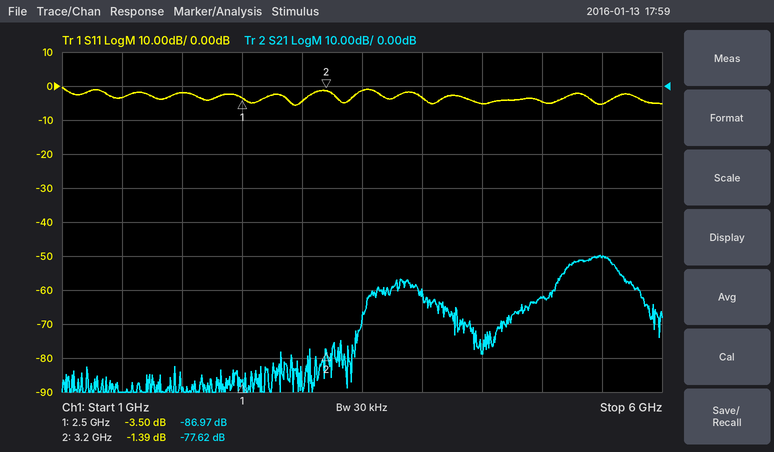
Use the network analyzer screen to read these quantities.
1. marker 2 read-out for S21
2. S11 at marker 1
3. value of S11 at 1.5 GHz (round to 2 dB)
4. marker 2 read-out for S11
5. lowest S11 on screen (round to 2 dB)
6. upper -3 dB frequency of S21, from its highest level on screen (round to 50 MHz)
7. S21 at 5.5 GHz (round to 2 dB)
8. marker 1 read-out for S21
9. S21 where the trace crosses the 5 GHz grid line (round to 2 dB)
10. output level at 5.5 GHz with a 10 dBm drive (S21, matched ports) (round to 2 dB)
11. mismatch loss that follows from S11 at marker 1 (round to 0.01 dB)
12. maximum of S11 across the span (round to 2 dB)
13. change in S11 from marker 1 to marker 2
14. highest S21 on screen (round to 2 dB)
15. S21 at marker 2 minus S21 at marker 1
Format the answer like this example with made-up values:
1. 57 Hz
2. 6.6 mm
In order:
1. -77.62 dB
2. -3.50 dB
3. -4 dB
4. -1.39 dB
5. -6 dB
6. 5.60 GHz
7. -50 dB
8. -86.97 dB
9. -62 dB
10. -40 dBm
11. 2.57 dB
12. 0 dB
13. 2.11 dB
14. -50 dB
15. 9.35 dB
